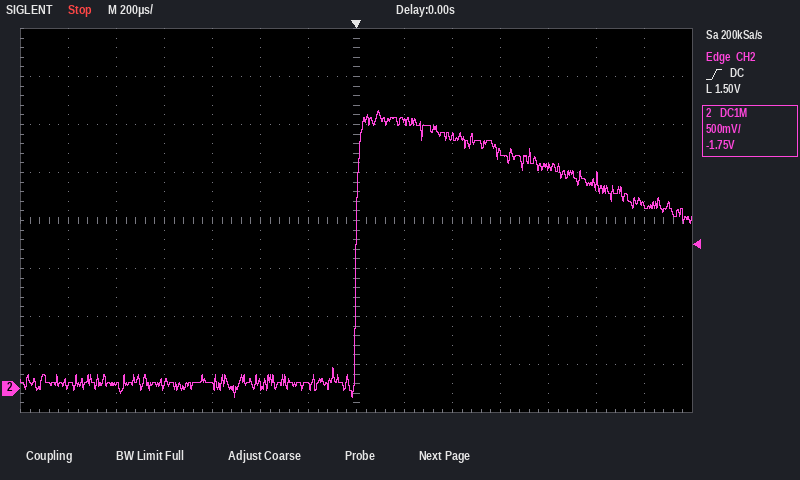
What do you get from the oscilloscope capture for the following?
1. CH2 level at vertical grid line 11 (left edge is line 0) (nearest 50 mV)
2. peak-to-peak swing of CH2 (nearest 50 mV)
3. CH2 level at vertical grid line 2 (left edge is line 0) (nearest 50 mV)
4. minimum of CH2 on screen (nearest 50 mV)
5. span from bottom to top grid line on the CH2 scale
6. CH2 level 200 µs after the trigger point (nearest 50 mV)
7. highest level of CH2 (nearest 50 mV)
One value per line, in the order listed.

2.30 V
3.00 V
50 mV
-100 mV
4 V
2.80 V
2.90 V
